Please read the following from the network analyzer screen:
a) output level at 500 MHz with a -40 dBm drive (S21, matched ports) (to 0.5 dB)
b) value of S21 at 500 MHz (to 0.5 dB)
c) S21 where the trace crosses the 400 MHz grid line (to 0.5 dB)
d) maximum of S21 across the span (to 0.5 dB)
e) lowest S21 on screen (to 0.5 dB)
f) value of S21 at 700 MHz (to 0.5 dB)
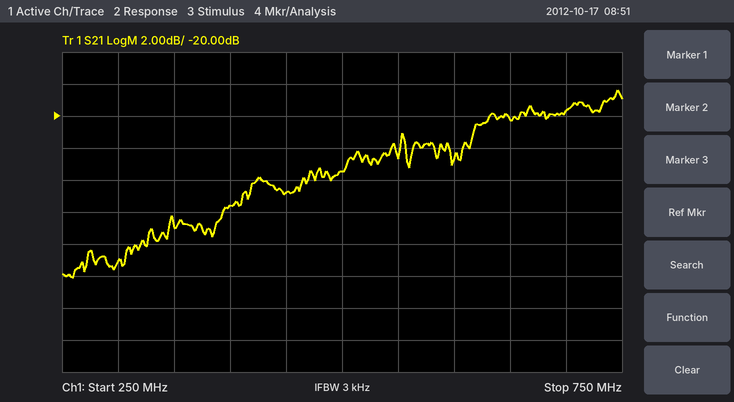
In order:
-63.5 dBm
-23.5 dB
-25.5 dB
-18.5 dB
-30.0 dB
-19.5 dB
